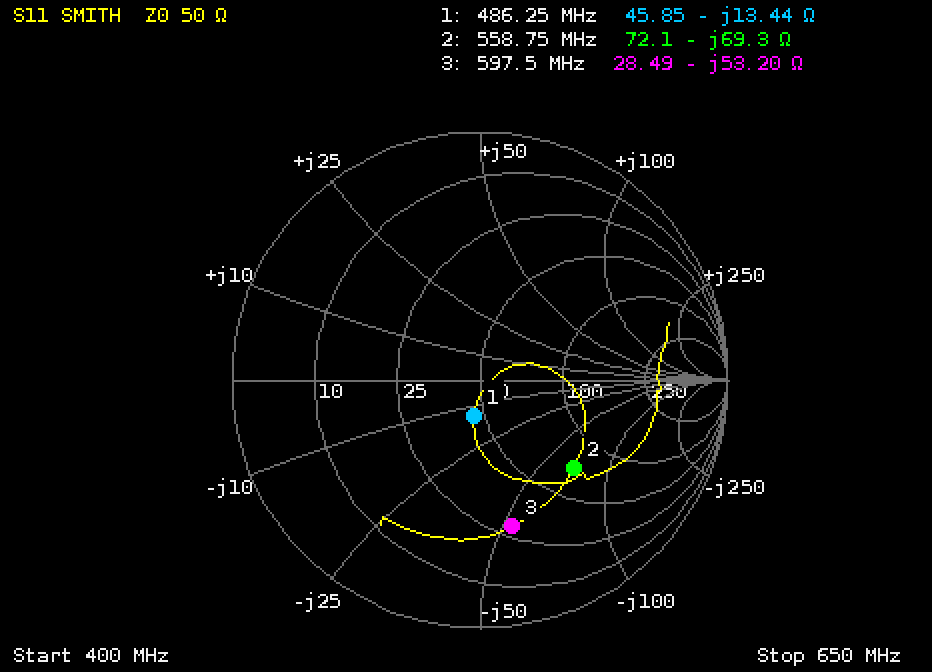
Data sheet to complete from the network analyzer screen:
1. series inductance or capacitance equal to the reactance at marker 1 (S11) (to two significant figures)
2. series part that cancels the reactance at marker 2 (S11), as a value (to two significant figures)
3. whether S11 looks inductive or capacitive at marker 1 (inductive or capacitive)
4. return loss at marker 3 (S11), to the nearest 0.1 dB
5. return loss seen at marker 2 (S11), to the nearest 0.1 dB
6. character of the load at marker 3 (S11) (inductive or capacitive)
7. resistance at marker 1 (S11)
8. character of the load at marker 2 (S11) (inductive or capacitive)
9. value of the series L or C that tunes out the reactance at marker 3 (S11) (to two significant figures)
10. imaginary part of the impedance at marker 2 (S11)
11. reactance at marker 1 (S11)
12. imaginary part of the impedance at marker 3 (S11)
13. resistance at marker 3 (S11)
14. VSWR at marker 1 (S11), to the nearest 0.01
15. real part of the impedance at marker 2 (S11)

24 pF
20 nH
capacitive
4.4 dB
5.7 dB
capacitive
45.85 Ω
capacitive
14 nH
-69.3 Ω
-13.44 Ω
-53.20 Ω
28.49 Ω
1.34
72.1 Ω
